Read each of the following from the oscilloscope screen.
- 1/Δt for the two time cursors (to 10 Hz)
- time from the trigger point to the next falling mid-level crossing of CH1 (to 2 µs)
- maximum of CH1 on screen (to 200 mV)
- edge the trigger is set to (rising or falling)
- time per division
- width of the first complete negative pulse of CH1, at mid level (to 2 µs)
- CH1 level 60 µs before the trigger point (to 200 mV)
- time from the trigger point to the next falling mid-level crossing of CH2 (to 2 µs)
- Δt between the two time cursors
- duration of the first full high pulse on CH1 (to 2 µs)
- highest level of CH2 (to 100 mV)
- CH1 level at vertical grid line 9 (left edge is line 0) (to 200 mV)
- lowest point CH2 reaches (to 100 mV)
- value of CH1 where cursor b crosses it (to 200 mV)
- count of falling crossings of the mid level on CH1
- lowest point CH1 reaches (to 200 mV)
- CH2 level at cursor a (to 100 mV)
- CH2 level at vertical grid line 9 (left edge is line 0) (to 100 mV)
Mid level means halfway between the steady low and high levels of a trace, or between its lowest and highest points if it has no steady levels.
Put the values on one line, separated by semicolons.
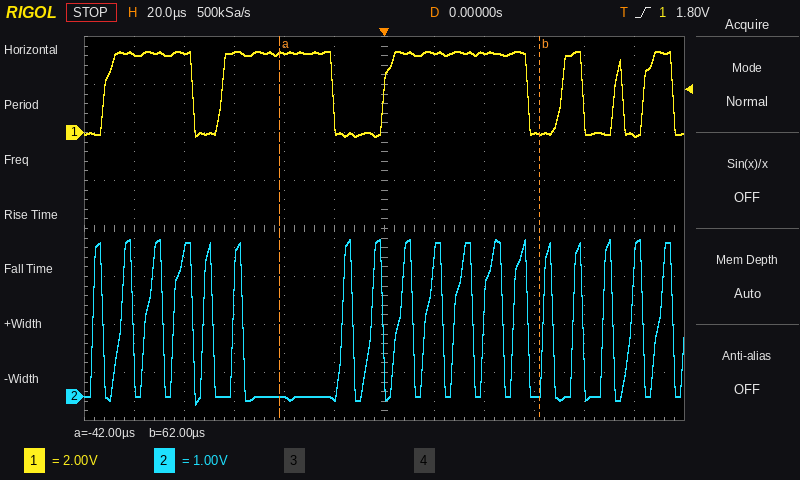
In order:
9.62 kHz; 58 µs; 3.4 V; rising; 20 µs; 12 µs; 3.4 V; 12 µs; 104 µs; 36 µs; 3.3 V; 0.0 V; -200 mV; 0.0 V; 6; -200 mV; 0.0 V; 0.0 V
